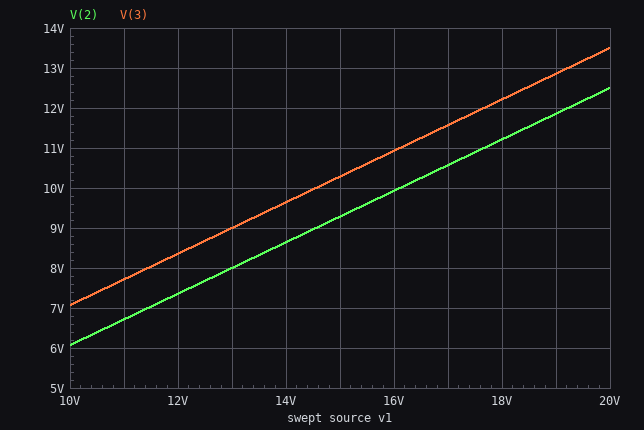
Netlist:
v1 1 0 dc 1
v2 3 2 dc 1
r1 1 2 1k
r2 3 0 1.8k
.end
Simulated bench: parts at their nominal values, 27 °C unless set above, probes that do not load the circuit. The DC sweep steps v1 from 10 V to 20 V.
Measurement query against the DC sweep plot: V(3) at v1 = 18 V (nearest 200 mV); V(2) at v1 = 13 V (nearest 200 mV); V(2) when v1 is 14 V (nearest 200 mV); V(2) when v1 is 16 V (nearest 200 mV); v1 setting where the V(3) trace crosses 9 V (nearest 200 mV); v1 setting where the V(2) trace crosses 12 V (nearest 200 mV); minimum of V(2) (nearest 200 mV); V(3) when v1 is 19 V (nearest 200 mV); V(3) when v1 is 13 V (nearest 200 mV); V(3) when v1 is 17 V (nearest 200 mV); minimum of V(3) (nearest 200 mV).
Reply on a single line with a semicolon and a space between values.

12.2 V; 8.0 V; 8.6 V; 10.0 V; 13.0 V; 19.2 V; 6.0 V; 12.8 V; 9.0 V; 11.6 V; 7.0 V
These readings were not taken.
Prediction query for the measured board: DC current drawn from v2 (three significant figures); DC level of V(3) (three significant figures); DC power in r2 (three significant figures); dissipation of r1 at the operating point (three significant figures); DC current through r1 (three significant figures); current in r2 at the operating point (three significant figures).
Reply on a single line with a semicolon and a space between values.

714 µA; 1.29 V; 918 µW; 510 µW; 714 µA; 714 µA
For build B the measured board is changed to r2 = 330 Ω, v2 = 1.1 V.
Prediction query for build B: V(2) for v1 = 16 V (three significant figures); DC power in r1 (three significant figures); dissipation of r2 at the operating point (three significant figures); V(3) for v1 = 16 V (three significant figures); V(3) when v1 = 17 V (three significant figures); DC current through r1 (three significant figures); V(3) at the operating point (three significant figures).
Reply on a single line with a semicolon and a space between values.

3.14 V; 2.49 mW; 823 µW; 4.24 V; 4.49 V; 1.58 mA; 521 mV
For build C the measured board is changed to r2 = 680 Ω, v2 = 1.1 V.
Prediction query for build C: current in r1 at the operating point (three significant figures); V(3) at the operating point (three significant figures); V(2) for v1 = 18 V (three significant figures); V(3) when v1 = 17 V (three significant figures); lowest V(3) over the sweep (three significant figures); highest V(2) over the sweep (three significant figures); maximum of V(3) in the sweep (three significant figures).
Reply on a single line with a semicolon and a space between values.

1.25 mA; 850 mV; 6.63 V; 7.33 V; 4.49 V; 7.44 V; 8.54 V
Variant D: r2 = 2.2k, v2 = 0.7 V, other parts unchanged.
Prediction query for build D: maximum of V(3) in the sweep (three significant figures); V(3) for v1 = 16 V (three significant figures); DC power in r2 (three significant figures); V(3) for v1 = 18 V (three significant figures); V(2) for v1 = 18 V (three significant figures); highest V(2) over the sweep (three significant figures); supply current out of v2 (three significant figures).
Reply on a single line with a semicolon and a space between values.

14.2 V; 11.5 V; 621 µW; 12.9 V; 12.2 V; 13.5 V; 531 µA
